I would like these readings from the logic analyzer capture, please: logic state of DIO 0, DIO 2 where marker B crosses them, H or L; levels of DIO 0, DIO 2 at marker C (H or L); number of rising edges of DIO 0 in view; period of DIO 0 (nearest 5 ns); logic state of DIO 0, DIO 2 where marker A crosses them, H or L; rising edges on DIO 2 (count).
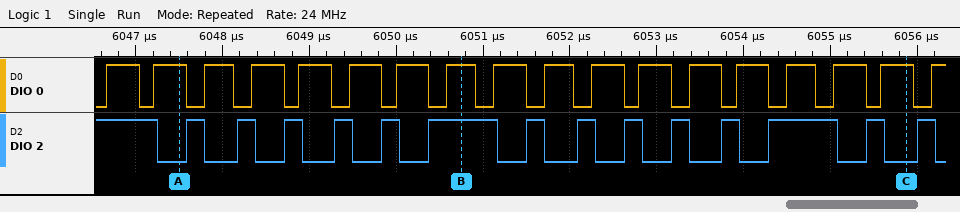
DIO 0=H, DIO 2=H
DIO 0=H, DIO 2=L
18
560 ns
DIO 0=H, DIO 2=L
14
